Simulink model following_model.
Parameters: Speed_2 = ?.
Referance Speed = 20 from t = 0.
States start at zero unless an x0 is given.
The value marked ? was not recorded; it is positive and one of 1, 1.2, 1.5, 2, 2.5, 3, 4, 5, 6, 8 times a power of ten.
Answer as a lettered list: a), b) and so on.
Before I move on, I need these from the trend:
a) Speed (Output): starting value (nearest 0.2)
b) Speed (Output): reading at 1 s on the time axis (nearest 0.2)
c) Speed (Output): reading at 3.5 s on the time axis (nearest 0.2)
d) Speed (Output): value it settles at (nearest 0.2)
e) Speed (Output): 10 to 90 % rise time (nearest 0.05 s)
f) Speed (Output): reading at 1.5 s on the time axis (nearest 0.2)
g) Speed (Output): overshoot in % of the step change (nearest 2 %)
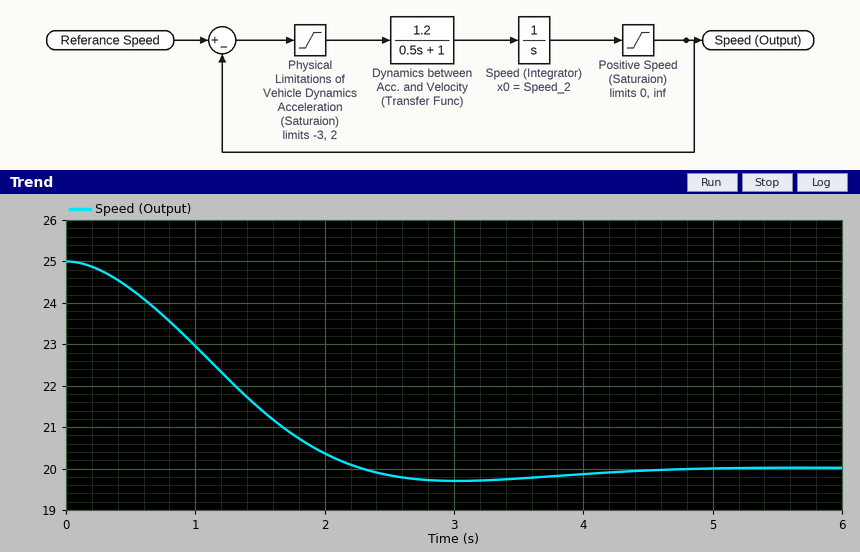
a) 25.0
b) 23.0
c) 19.8
d) 20.0
e) 1.50 s
f) 21.4
g) 6 %
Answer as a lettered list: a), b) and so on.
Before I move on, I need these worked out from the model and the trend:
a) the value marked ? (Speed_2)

a) 25
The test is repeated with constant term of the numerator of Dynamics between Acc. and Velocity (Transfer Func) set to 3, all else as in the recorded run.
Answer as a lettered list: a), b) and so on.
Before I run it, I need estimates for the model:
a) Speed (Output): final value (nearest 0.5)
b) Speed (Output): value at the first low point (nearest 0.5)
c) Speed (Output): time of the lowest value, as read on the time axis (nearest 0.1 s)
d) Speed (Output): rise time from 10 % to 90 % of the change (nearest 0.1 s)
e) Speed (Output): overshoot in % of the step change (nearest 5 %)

a) 20.0
b) 19.0
c) 1.6 s
d) 0.7 s
e) 20 %
